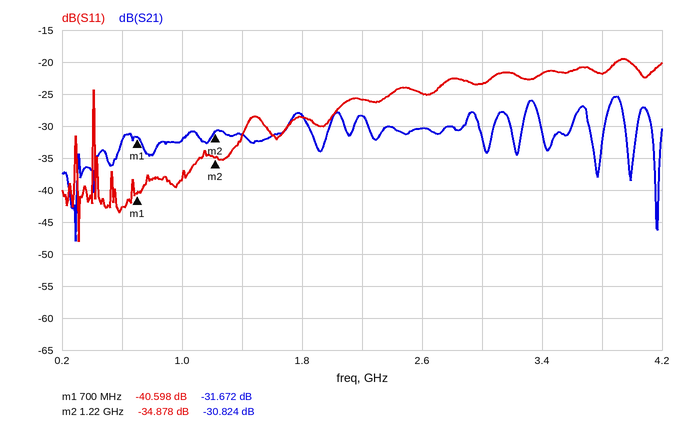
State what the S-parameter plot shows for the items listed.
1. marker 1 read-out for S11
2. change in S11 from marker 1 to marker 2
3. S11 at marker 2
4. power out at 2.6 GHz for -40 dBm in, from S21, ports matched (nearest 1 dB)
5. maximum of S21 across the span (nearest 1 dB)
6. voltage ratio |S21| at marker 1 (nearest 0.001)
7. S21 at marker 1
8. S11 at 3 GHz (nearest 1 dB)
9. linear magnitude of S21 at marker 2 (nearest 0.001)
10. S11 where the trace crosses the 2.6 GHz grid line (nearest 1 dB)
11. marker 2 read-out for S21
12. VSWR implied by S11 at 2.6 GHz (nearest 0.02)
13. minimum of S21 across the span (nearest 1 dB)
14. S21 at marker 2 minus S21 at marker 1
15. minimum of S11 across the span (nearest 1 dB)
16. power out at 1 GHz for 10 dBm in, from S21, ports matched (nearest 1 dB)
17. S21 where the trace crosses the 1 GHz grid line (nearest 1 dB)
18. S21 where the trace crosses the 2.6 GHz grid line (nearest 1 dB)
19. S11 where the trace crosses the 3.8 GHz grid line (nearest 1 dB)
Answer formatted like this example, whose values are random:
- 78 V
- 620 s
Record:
- -40.598 dB
- 5.720 dB
- -34.878 dB
- -70 dBm
- -25 dB
- 0.026
- -31.672 dB
- -23 dB
- 0.029
- -25 dB
- -30.824 dB
- 1.12
- -48 dB
- 0.848 dB
- -48 dB
- -22 dBm
- -32 dB
- -30 dB
- -22 dB
